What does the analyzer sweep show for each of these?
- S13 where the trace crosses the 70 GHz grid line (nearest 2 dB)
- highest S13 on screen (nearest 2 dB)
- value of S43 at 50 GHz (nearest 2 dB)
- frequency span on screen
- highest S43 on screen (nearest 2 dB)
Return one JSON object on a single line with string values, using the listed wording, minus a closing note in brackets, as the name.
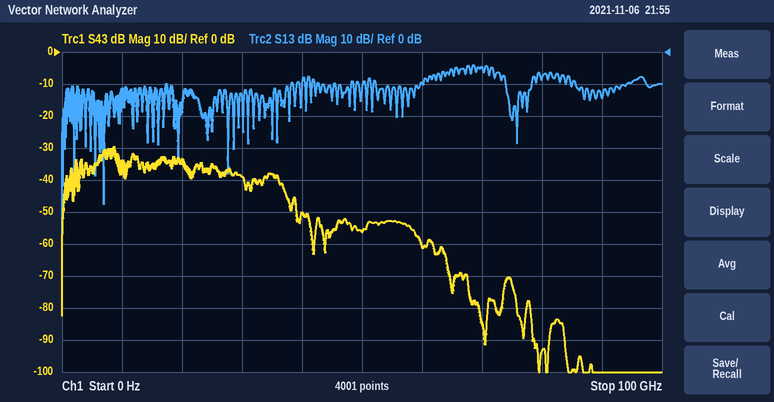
{"S13 where the trace crosses the 70 GHz grid line": "-4 dB", "highest S13 on screen": "-4 dB", "value of S43 at 50 GHz": "-56 dB", "frequency span on screen": "100 GHz", "highest S43 on screen": "-30 dB"}
